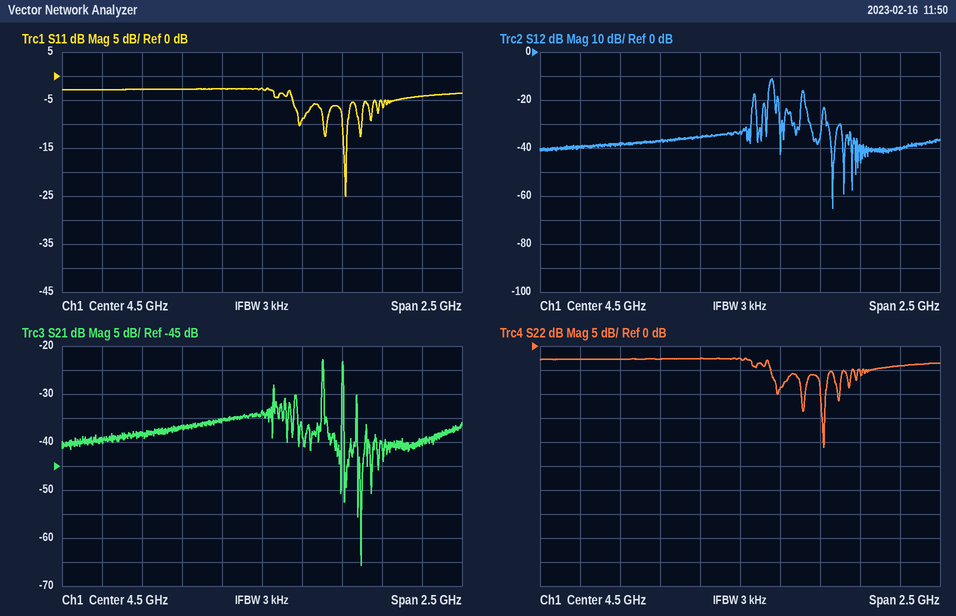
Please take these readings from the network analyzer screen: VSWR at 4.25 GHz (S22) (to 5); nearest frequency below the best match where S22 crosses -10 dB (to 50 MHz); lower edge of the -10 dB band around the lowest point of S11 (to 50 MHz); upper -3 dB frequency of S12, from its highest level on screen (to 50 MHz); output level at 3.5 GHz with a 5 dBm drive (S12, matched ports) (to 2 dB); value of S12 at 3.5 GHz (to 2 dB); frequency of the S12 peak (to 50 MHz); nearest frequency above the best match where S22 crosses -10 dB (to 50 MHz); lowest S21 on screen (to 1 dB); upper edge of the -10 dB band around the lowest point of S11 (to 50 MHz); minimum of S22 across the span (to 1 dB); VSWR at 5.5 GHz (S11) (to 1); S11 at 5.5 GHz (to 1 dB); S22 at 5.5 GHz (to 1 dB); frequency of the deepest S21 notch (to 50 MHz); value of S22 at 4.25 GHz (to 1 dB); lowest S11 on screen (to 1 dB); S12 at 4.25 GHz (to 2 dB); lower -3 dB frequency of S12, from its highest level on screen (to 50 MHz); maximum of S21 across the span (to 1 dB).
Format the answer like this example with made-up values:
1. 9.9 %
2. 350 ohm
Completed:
1. 5
2. 5.00 GHz
3. 5.00 GHz
4. 4.70 GHz
5. -34 dBm
6. -40 dB
7. 4.70 GHz
8. 5.05 GHz
9. -66 dB
10. 5.05 GHz
11. -21 dB
12. 4
13. -4 dB
14. -4 dB
15. 5.10 GHz
16. -3 dB
17. -25 dB
18. -36 dB
19. 4.70 GHz
20. -23 dB
